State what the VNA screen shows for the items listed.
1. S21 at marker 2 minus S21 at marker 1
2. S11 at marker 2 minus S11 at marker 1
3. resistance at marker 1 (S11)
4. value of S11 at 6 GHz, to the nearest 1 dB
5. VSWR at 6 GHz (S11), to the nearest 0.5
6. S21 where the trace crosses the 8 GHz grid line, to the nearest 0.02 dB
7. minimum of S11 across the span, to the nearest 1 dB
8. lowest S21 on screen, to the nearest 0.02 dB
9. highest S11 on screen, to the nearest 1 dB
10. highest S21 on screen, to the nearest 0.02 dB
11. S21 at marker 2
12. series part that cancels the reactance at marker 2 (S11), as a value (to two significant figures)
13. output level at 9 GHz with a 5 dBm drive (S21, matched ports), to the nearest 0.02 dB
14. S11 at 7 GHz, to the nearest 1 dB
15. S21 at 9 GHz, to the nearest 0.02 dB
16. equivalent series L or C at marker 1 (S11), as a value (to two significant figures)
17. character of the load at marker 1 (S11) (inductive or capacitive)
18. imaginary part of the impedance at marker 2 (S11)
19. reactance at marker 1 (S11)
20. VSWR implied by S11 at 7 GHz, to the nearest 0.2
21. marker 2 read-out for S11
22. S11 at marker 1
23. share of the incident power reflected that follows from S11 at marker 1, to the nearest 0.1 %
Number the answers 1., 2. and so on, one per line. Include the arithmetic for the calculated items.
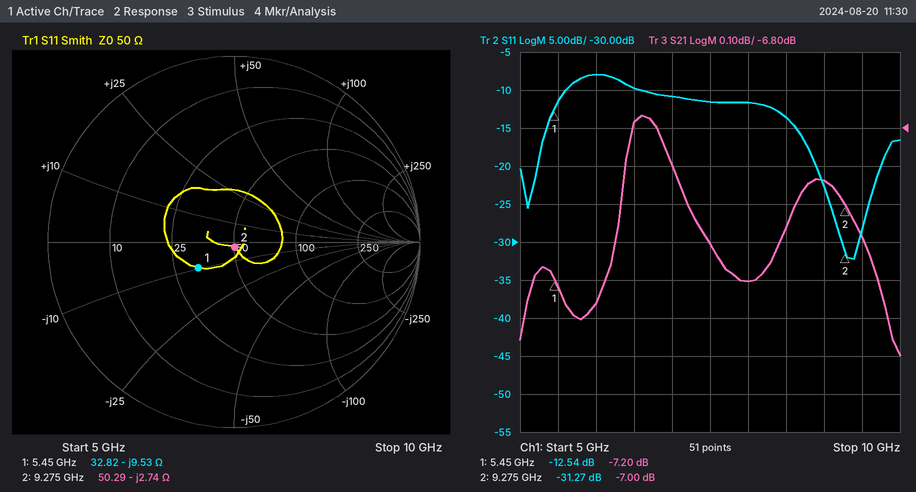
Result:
1. -7 − (-7.2) = 0.20 dB
2. -31.27 − (-12.54) = -18.73 dB
3. 32.82 Ω
4. -8 dB
5. |Γ| = 10^(-8/20) = 0.3981; VSWR = (1 + 0.3981)/(1 − 0.3981) ≈ 2.32, so 2.5 to the nearest 0.5
6. -7.20 dB
7. -32 dB
8. -7.40 dB
9. -8 dB
10. -6.76 dB
11. -7.00 dB
12. L = 2.74 Ω/(2π × 9.275 GHz) ≈ 47 pH
13. 5 dBm + (-6.94 dB) = -1.94 dBm
14. -11 dB
15. -6.94 dB
16. C = 1/(2π × 5.45 GHz × 9.53 Ω) ≈ 3.1 pF
17. capacitive
18. -2.74 Ω
19. -9.53 Ω
20. |Γ| = 10^(-11/20) = 0.2818; VSWR = (1 + 0.2818)/(1 − 0.2818) ≈ 1.8
21. -31.27 dB
22. -12.54 dB
23. 10^(-12.54/10) ≈ 5.6 %
